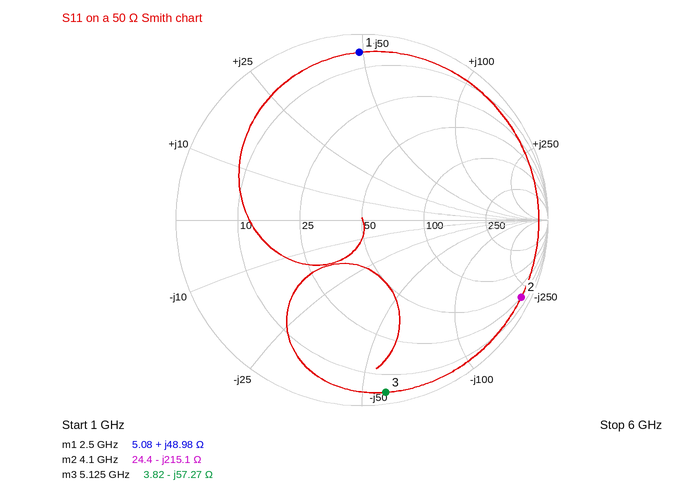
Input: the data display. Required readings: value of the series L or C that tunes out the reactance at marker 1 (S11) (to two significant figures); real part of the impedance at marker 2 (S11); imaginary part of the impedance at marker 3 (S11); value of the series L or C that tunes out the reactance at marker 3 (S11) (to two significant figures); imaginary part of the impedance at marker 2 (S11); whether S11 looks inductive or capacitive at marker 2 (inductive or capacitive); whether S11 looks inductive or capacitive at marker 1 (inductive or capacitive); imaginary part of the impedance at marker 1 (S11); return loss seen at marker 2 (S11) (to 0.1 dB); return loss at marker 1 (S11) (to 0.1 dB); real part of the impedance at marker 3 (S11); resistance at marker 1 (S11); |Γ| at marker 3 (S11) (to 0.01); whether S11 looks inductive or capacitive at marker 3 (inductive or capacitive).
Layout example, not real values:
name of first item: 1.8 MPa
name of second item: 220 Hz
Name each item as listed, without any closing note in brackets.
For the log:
value of the series L or C that tunes out the reactance at marker 1 (S11): 1.3 pF
real part of the impedance at marker 2: 24.4 Ω
imaginary part of the impedance at marker 3: -57.27 Ω
value of the series L or C that tunes out the reactance at marker 3 (S11): 1.8 nH
imaginary part of the impedance at marker 2: -215.1 Ω
whether S11 looks inductive or capacitive at marker 2: capacitive
whether S11 looks inductive or capacitive at marker 1: inductive
imaginary part of the impedance at marker 1: +48.98 Ω
return loss seen at marker 2 (S11): 0.4 dB
return loss at marker 1 (S11): 0.9 dB
real part of the impedance at marker 3: 3.82 Ω
resistance at marker 1: 5.08 Ω
|Γ| at marker 3 (S11): 0.94
whether S11 looks inductive or capacitive at marker 3: capacitive
